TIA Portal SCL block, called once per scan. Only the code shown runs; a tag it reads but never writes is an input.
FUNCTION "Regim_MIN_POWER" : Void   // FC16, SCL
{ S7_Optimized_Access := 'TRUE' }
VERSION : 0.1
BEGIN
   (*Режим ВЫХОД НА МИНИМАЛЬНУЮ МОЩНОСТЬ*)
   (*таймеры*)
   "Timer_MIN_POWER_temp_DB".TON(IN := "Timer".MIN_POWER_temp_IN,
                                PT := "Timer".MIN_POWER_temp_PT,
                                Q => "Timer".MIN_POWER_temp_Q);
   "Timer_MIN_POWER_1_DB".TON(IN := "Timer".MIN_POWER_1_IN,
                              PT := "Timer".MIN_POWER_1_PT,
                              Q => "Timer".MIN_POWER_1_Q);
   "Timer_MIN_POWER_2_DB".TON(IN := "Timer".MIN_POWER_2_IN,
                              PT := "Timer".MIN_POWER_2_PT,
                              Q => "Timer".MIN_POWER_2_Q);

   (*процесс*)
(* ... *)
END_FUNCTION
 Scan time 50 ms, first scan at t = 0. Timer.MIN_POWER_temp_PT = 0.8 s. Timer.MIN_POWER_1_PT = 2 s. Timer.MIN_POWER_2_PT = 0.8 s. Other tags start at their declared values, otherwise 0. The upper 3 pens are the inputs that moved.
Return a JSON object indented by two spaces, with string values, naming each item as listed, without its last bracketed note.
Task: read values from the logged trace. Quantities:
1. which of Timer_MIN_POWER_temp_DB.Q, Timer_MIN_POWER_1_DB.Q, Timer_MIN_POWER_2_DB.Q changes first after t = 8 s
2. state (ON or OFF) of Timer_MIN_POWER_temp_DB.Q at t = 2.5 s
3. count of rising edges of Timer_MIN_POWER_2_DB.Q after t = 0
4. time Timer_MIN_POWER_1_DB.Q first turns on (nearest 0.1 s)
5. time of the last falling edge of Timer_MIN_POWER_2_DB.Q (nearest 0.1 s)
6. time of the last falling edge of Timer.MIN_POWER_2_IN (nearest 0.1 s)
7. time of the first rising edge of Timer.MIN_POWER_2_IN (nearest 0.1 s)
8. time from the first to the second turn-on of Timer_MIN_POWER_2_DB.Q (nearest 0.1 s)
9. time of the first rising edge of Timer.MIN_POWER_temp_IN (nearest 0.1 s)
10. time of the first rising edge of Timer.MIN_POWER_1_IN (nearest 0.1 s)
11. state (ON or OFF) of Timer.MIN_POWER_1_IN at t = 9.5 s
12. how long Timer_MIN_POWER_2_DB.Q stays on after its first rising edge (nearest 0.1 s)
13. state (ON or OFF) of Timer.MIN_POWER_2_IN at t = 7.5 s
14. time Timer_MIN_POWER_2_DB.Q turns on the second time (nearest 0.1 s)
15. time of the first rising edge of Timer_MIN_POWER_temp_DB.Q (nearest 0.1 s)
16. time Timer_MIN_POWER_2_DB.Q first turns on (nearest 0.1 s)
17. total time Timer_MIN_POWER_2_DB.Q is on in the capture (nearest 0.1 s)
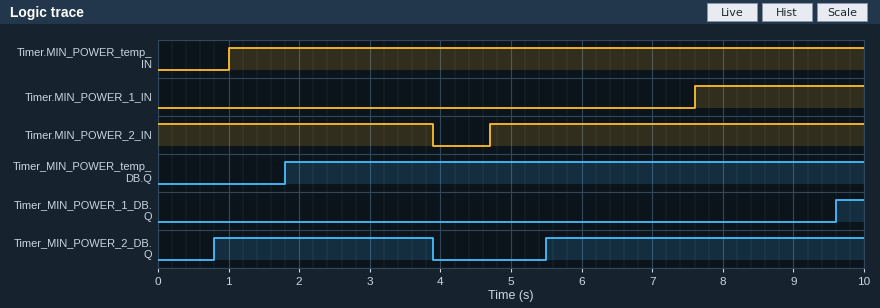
{
  "which of Timer_MIN_POWER_temp_DB.Q, Timer_MIN_POWER_1_DB.Q, Timer_MIN_POWER_2_DB.Q changes first after t = 8 s": "Timer_MIN_POWER_1_DB.Q",
  "state (ON or OFF) of Timer_MIN_POWER_temp_DB.Q at t = 2.5 s": "ON",
  "count of rising edges of Timer_MIN_POWER_2_DB.Q after t = 0": "2",
  "time Timer_MIN_POWER_1_DB.Q first turns on": "9.6 s",
  "time of the last falling edge of Timer_MIN_POWER_2_DB.Q": "3.9 s",
  "time of the last falling edge of Timer.MIN_POWER_2_IN": "3.9 s",
  "time of the first rising edge of Timer.MIN_POWER_2_IN": "4.7 s",
  "time from the first to the second turn-on of Timer_MIN_POWER_2_DB.Q": "4.7 s",
  "time of the first rising edge of Timer.MIN_POWER_temp_IN": "1.0 s",
  "time of the first rising edge of Timer.MIN_POWER_1_IN": "7.6 s",
  "state (ON or OFF) of Timer.MIN_POWER_1_IN at t = 9.5 s": "ON",
  "how long Timer_MIN_POWER_2_DB.Q stays on after its first rising edge": "3.1 s",
  "state (ON or OFF) of Timer.MIN_POWER_2_IN at t = 7.5 s": "ON",
  "time Timer_MIN_POWER_2_DB.Q turns on the second time": "5.5 s",
  "time of the first rising edge of Timer_MIN_POWER_temp_DB.Q": "1.8 s",
  "time Timer_MIN_POWER_2_DB.Q first turns on": "0.8 s",
  "total time Timer_MIN_POWER_2_DB.Q is on in the capture": "7.6 s"
}
